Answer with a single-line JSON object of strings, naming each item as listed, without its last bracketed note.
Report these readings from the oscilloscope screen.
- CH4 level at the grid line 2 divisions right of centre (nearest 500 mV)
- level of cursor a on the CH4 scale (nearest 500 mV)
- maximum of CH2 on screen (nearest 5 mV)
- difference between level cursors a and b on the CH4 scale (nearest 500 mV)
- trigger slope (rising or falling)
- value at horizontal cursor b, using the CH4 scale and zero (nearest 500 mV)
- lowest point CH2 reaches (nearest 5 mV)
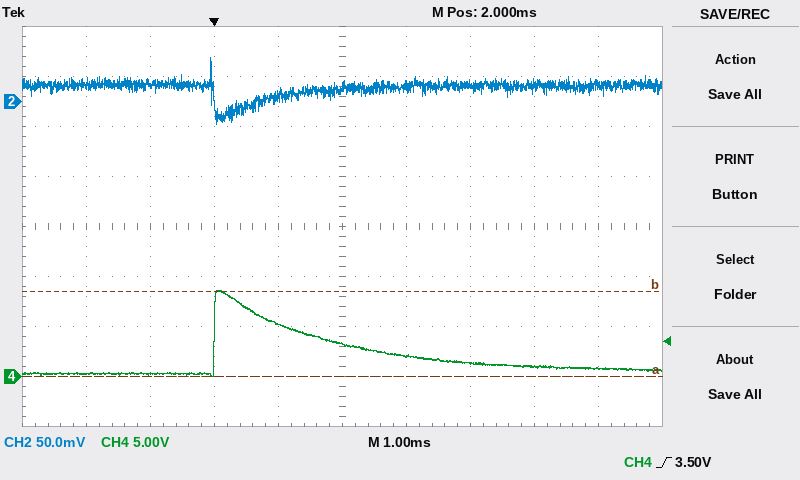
{"CH4 level at the grid line 2 divisions right of centre": "1.5 V", "level of cursor a on the CH4 scale": "0.0 V", "maximum of CH2 on screen": "45 mV", "difference between level cursors a and b on the CH4 scale": "8.5 V", "trigger slope": "rising", "value at horizontal cursor b, using the CH4 scale and zero": "8.5 V", "lowest point CH2 reaches": "-25 mV"}
